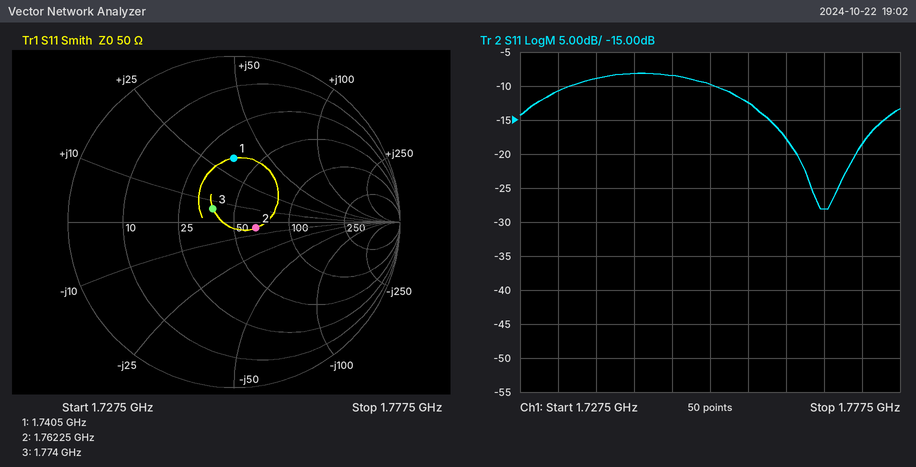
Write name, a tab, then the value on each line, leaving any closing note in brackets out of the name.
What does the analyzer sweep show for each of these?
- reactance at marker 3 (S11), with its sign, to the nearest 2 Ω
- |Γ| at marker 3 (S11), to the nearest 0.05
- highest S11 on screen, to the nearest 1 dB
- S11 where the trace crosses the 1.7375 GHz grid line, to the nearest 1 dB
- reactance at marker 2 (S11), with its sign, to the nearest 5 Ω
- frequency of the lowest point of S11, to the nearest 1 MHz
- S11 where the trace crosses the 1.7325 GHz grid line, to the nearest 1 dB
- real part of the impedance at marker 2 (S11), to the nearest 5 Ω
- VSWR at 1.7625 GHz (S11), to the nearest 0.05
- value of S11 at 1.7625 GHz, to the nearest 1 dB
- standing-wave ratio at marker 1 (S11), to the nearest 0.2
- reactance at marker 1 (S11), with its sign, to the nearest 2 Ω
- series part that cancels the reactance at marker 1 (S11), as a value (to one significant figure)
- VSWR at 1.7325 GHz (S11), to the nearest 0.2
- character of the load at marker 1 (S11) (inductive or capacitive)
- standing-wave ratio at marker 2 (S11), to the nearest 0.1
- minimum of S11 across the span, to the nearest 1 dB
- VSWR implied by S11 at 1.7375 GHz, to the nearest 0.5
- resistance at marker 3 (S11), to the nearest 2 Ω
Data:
reactance at marker 3 (S11), with its sign, to the nearest 2 Ω	+6 Ω
|Γ| at marker 3 (S11), to the nearest 0.05	0.15
highest S11 on screen, to the nearest 1 dB	-8 dB
S11 where the trace crosses the 1.7375 GHz grid line, to the nearest 1 dB	-9 dB
reactance at marker 2 (S11), with its sign, to the nearest 5 Ω	-5 Ω
frequency of the lowest point of S11, to the nearest 1 MHz	1.768 GHz
S11 where the trace crosses the 1.7325 GHz grid line, to the nearest 1 dB	-11 dB
real part of the impedance at marker 2 (S11), to the nearest 5 Ω	65 Ω
VSWR at 1.7625 GHz (S11), to the nearest 0.05	1.30
value of S11 at 1.7625 GHz, to the nearest 1 dB	-18 dB
standing-wave ratio at marker 1 (S11), to the nearest 0.2	2.2
reactance at marker 1 (S11), with its sign, to the nearest 2 Ω	+34 Ω
series part that cancels the reactance at marker 1 (S11), as a value	3 pF
VSWR at 1.7325 GHz (S11), to the nearest 0.2	1.8
character of the load at marker 1 (S11)	inductive
standing-wave ratio at marker 2 (S11), to the nearest 0.1	1.3
minimum of S11 across the span, to the nearest 1 dB	-28 dB
VSWR implied by S11 at 1.7375 GHz, to the nearest 0.5	2.0
resistance at marker 3 (S11), to the nearest 2 Ω	38 Ω
